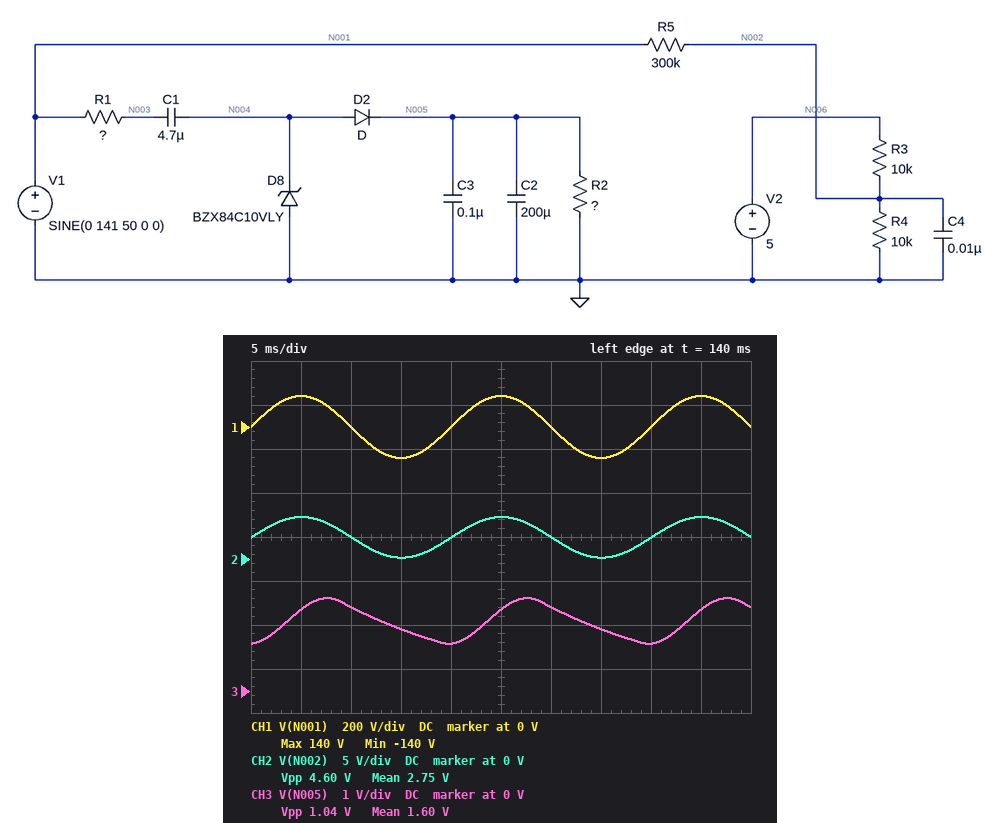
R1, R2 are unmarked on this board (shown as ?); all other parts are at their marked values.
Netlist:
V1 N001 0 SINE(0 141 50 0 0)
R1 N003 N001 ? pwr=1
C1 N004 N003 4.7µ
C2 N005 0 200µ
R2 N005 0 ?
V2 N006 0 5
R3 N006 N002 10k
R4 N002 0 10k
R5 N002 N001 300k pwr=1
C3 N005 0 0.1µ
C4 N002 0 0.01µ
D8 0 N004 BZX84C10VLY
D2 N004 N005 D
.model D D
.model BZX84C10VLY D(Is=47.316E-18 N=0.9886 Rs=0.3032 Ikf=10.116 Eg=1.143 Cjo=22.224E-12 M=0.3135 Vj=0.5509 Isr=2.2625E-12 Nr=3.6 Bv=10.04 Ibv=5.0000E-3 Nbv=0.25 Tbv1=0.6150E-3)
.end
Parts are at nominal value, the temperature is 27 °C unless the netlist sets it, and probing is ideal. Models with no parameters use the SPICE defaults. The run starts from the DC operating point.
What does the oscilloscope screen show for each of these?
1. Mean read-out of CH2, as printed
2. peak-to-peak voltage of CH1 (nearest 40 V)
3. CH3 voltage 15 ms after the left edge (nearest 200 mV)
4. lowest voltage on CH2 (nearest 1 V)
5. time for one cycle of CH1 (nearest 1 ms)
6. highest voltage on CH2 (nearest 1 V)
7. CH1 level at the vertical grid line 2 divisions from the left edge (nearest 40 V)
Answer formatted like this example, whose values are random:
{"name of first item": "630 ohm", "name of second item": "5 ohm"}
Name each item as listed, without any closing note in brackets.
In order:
{"Mean read-out of CH2, as printed": "2.75 V", "peak-to-peak voltage of CH1": "280 V", "CH3 voltage 15 ms after the left edge": "1.4 V", "lowest voltage on CH2": "0 V", "time for one cycle of CH1": "20 ms", "highest voltage on CH2": "5 V", "CH1 level at the vertical grid line 2 divisions from the left edge": "0 V"}
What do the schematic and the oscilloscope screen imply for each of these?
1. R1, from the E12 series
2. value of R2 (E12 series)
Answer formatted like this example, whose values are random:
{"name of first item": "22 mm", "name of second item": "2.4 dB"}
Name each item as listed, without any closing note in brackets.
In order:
{"R1, from the E12 series": "2.2 kΩ", "value of R2": "82 Ω"}
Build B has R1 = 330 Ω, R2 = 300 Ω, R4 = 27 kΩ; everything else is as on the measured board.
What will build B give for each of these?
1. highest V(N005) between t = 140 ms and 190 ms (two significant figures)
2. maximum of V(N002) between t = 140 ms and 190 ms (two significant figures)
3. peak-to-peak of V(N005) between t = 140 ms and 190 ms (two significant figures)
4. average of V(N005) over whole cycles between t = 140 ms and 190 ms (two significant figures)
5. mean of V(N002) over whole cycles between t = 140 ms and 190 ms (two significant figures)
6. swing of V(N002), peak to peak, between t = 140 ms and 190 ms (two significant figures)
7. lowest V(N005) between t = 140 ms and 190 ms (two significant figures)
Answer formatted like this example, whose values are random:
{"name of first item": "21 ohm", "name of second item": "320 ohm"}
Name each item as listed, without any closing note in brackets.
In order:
{"highest V(N005) between t = 140 ms and 190 ms": "9.4 V", "maximum of V(N002) between t = 140 ms and 190 ms": "6.9 V", "peak-to-peak of V(N005) between t = 140 ms and 190 ms": "1.6 V", "average of V(N005) over whole cycles between t = 140 ms and 190 ms": "8.7 V", "mean of V(N002) over whole cycles between t = 140 ms and 190 ms": "3.6 V", "swing of V(N002), peak to peak, between t = 140 ms and 190 ms": "6.7 V", "lowest V(N005) between t = 140 ms and 190 ms": "7.8 V"}
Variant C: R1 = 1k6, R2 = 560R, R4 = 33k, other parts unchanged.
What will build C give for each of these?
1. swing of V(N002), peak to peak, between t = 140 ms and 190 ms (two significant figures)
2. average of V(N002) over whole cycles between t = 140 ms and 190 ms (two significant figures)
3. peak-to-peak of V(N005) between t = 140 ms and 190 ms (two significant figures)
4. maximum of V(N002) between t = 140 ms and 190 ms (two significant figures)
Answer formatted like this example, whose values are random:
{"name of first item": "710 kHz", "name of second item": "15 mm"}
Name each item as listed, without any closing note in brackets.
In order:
{"swing of V(N002), peak to peak, between t = 140 ms and 190 ms": "7.0 V", "average of V(N002) over whole cycles between t = 140 ms and 190 ms": "3.7 V", "peak-to-peak of V(N005) between t = 140 ms and 190 ms": "890 mV", "maximum of V(N002) between t = 140 ms and 190 ms": "7.3 V"}
